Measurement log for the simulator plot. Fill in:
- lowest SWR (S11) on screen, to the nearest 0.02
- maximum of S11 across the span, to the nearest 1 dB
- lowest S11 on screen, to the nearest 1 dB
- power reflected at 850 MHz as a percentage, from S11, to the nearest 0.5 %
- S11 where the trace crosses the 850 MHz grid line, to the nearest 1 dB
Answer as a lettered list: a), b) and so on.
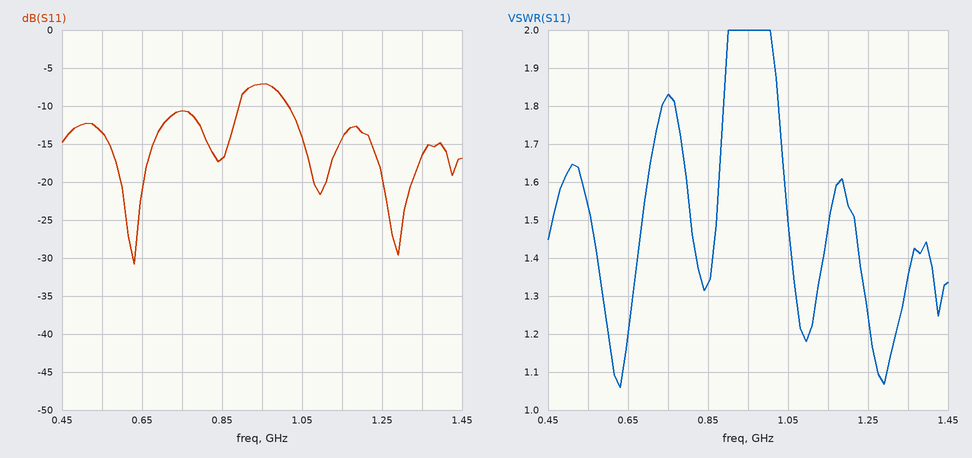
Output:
a) 1.06
b) -7 dB
c) -31 dB
d) 2.0 %
e) -17 dB
